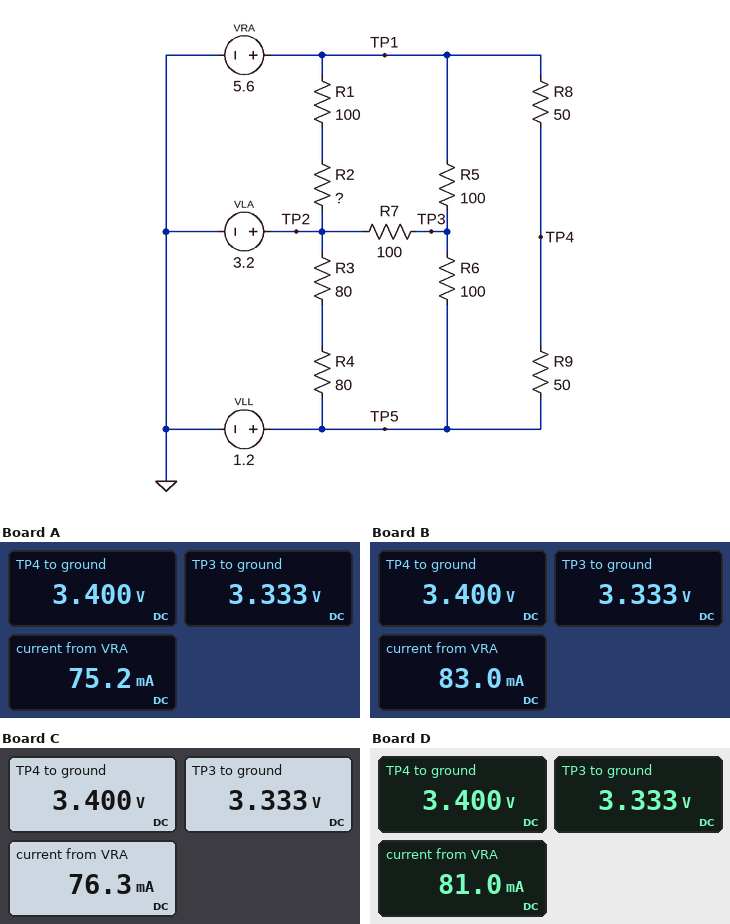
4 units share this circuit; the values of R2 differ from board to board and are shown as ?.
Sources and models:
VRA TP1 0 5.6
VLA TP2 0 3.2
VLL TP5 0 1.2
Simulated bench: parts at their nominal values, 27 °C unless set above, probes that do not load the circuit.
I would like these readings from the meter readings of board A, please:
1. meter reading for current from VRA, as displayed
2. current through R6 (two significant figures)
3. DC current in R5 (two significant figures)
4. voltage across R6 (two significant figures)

75.2 mA
21 mA
23 mA
2.1 V
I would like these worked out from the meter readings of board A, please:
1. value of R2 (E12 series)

180 Ω
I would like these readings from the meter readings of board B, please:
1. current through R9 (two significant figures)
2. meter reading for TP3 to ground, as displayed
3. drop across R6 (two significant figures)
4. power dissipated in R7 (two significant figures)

44 mA
3.333 V
2.1 V
180 µW
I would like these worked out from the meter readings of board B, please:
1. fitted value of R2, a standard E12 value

47 Ω
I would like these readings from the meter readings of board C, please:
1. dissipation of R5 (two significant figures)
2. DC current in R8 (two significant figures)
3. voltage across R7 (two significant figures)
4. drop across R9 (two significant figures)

51 mW
44 mA
130 mV
2.2 V
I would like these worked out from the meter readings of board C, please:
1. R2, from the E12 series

150 Ω
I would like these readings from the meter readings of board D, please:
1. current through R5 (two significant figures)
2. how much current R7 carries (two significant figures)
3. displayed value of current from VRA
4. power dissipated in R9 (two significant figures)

23 mA
1.3 mA
81.0 mA
97 mW
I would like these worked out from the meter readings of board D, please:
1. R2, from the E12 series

68 Ω
